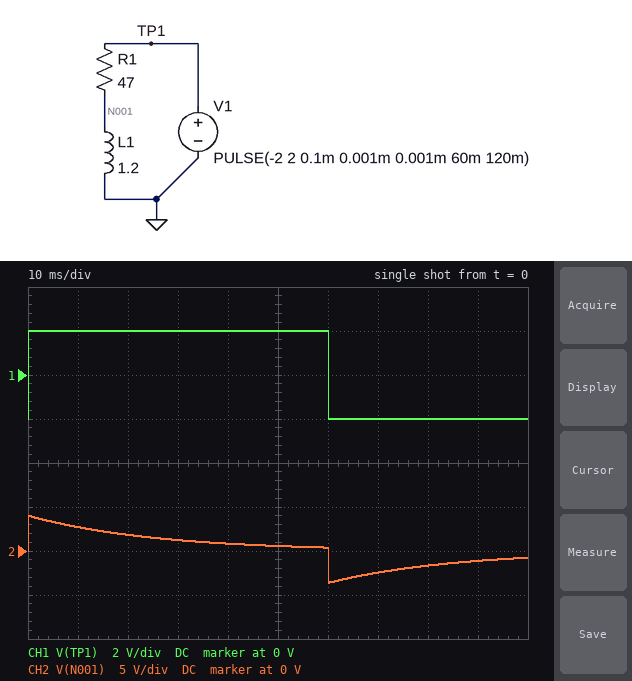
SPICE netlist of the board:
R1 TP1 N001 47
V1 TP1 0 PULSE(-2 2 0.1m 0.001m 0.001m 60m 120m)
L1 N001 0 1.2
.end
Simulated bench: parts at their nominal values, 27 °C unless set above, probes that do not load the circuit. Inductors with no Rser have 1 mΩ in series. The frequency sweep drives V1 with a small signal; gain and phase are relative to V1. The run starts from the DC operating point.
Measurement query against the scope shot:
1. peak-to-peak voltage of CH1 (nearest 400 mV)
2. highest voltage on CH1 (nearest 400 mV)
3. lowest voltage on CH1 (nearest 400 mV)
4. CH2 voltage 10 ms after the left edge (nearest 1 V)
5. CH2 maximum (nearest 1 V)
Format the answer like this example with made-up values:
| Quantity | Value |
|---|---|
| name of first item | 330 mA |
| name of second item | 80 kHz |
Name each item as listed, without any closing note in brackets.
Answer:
| Quantity | Value |
|---|---|
| peak-to-peak voltage of CH1 | 4.0 V |
| highest voltage on CH1 | 2.0 V |
| lowest voltage on CH1 | -2.0 V |
| CH2 voltage 10 ms after the left edge | 3 V |
| CH2 maximum | 4 V |
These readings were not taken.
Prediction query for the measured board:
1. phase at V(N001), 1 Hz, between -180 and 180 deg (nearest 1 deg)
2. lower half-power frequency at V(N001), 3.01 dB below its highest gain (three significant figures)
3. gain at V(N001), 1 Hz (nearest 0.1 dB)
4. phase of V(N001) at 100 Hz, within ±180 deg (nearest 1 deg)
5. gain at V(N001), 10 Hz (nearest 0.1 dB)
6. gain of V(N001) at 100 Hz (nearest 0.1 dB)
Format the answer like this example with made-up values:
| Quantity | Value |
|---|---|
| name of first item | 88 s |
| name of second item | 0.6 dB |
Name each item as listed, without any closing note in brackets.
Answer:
| Quantity | Value |
|---|---|
| phase at V(N001), 1 Hz, between -180 and 180 deg | 81 deg |
| lower half-power frequency at V(N001), 3.01 dB below its highest gain | 6.23 Hz |
| gain at V(N001), 1 Hz | -16.0 dB |
| phase of V(N001) at 100 Hz, within ±180 deg | 4 deg |
| gain at V(N001), 10 Hz | -1.4 dB |
| gain of V(N001) at 100 Hz | 0 dB |
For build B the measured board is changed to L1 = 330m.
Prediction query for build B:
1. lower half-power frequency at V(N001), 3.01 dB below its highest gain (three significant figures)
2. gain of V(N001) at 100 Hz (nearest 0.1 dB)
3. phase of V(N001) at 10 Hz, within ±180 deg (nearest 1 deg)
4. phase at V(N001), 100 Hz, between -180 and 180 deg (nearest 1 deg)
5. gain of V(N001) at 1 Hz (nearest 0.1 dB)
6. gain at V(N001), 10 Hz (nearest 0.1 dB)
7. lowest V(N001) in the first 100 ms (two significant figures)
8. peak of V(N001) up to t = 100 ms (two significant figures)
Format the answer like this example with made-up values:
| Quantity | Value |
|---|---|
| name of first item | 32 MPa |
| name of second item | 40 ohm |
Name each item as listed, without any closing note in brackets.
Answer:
| Quantity | Value |
|---|---|
| lower half-power frequency at V(N001), 3.01 dB below its highest gain | 22.7 Hz |
| gain of V(N001) at 100 Hz | -0.2 dB |
| phase of V(N001) at 10 Hz, within ±180 deg | 66 deg |
| phase at V(N001), 100 Hz, between -180 and 180 deg | 13 deg |
| gain of V(N001) at 1 Hz | -27.1 dB |
| gain at V(N001), 10 Hz | -7.9 dB |
| lowest V(N001) in the first 100 ms | -4.0 V |
| peak of V(N001) up to t = 100 ms | 4.0 V |
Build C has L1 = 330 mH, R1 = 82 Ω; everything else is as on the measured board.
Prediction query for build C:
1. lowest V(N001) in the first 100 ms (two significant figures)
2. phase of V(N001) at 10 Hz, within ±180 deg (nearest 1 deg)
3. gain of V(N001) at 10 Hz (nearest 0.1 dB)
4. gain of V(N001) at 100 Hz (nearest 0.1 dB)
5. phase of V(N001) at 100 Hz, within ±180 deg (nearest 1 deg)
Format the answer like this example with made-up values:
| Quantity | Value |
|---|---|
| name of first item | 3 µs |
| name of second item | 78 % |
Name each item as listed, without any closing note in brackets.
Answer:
| Quantity | Value |
|---|---|
| lowest V(N001) in the first 100 ms | -4.0 V |
| phase of V(N001) at 10 Hz, within ±180 deg | 76 deg |
| gain of V(N001) at 10 Hz | -12.2 dB |
| gain of V(N001) at 100 Hz | -0.6 dB |
| phase of V(N001) at 100 Hz, within ±180 deg | 22 deg |
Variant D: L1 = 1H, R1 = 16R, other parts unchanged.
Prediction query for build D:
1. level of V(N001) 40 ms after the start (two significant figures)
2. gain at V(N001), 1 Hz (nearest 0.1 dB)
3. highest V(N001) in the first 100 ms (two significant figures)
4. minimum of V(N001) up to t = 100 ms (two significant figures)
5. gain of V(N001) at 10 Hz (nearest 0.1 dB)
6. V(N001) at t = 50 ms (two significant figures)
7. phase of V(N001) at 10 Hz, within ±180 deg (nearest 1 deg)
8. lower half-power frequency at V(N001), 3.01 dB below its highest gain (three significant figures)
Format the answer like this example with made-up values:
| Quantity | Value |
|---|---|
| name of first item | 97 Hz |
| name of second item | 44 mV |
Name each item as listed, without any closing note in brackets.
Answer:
| Quantity | Value |
|---|---|
| level of V(N001) 40 ms after the start | 2.1 V |
| gain at V(N001), 1 Hz | -8.7 dB |
| highest V(N001) in the first 100 ms | 4.0 V |
| minimum of V(N001) up to t = 100 ms | -2.5 V |
| gain of V(N001) at 10 Hz | -0.3 dB |
| V(N001) at t = 50 ms | 1.8 V |
| phase of V(N001) at 10 Hz, within ±180 deg | 14 deg |
| lower half-power frequency at V(N001), 3.01 dB below its highest gain | 2.55 Hz |
